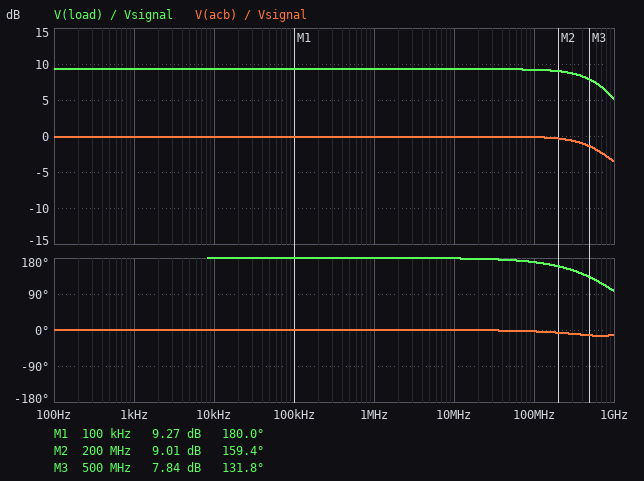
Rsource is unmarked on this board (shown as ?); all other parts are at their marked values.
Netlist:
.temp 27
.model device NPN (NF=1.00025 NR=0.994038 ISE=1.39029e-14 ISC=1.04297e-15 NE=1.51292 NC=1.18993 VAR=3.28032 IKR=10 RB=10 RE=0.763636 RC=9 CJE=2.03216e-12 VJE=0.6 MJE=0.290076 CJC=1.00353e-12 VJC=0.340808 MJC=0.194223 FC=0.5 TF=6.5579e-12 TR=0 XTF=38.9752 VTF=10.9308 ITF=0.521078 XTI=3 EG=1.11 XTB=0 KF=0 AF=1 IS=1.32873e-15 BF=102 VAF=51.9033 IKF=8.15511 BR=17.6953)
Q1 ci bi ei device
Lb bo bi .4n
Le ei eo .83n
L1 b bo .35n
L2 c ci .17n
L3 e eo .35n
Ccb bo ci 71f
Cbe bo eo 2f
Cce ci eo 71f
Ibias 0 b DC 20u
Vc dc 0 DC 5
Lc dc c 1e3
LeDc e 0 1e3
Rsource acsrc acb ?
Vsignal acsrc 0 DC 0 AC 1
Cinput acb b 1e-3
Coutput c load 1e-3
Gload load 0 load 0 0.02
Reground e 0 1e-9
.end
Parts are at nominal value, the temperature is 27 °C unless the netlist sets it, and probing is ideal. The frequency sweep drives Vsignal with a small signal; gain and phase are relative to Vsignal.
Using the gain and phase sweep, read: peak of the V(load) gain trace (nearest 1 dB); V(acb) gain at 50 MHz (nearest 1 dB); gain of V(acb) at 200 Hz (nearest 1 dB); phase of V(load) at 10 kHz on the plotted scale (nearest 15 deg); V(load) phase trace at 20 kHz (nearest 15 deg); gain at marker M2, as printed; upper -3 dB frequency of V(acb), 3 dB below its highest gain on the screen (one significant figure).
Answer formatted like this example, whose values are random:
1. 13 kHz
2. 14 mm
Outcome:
1. 9 dB
2. 0 dB
3. 0 dB
4. 180 deg
5. 180 deg
6. 9.01 dB
7. 900 MHz
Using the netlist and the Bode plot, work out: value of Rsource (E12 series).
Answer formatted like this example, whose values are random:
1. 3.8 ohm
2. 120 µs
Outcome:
1. 15 Ω
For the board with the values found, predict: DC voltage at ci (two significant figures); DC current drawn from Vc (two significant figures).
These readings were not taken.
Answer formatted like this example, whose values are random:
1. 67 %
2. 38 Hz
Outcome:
1. 5.0 V
2. 1.6 mA
